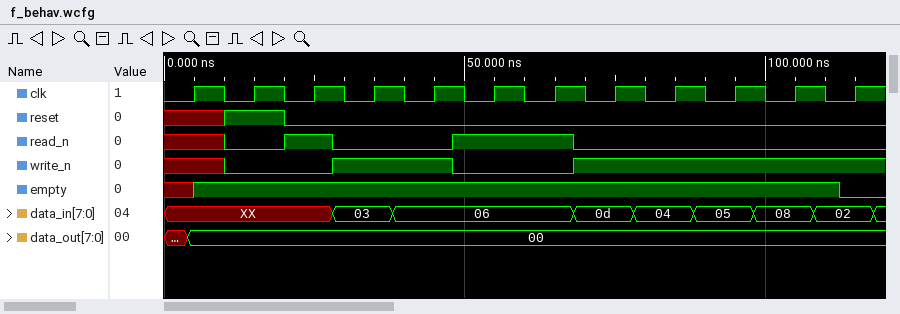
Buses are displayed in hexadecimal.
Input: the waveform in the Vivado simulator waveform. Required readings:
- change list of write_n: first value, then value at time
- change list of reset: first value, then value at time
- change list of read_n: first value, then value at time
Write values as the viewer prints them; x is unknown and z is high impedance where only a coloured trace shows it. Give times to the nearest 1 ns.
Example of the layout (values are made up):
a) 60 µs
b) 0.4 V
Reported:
a) x, 0 at 10 ns, 1 at 28 ns, 0 at 48 ns, 1 at 68 ns
b) x, 1 at 10 ns, 0 at 20 ns
c) x, 0 at 10 ns, 1 at 20 ns, 0 at 28 ns, 1 at 48 ns, 0 at 68 ns
